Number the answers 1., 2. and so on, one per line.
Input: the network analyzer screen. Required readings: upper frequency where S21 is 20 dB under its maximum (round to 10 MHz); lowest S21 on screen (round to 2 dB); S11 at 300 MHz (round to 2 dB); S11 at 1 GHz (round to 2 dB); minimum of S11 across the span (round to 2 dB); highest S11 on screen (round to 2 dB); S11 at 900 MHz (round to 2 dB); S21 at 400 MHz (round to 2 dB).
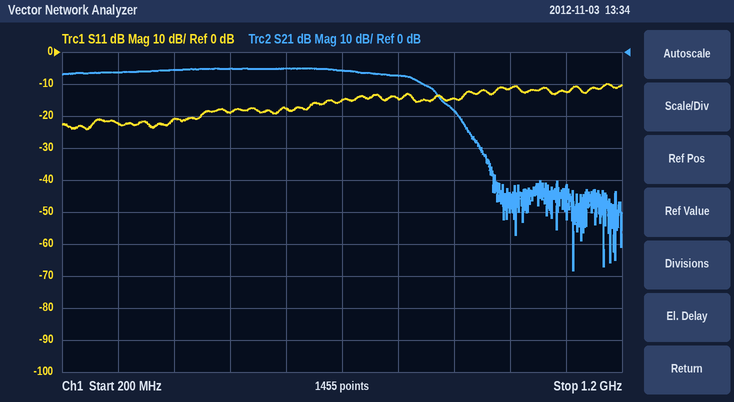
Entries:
1. 930 MHz
2. -68 dB
3. -22 dB
4. -12 dB
5. -24 dB
6. -10 dB
7. -14 dB
8. -6 dB
